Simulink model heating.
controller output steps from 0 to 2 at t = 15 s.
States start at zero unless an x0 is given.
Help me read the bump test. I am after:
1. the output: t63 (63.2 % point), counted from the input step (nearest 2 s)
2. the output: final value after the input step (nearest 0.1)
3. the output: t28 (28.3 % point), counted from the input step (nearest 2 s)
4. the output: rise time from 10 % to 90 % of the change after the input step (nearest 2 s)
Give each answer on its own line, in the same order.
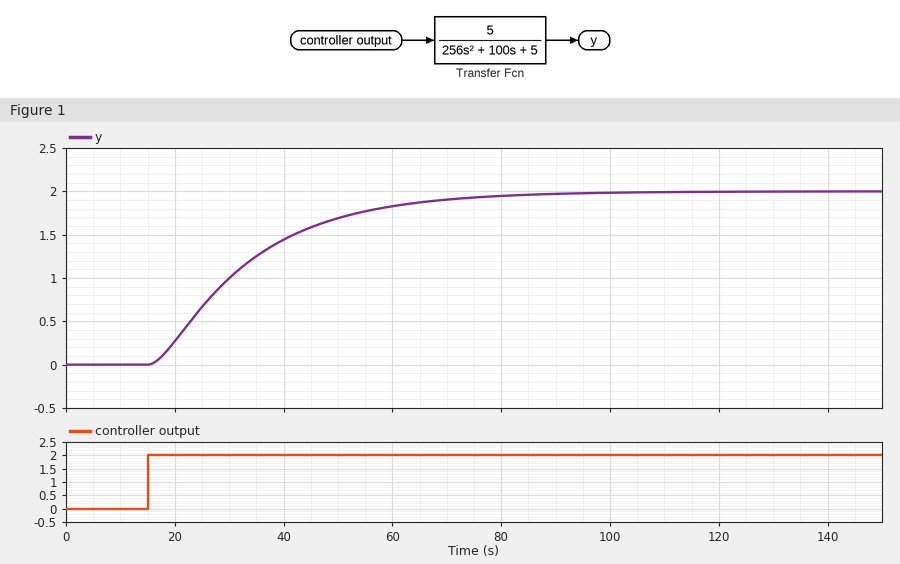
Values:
20 s
2.0
8 s
38 s
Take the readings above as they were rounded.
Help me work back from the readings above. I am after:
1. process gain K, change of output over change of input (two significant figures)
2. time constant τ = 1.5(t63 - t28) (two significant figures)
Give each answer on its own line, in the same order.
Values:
1.0
18 s
